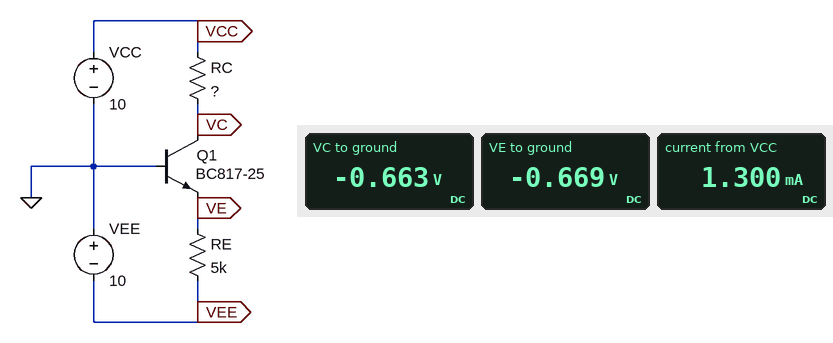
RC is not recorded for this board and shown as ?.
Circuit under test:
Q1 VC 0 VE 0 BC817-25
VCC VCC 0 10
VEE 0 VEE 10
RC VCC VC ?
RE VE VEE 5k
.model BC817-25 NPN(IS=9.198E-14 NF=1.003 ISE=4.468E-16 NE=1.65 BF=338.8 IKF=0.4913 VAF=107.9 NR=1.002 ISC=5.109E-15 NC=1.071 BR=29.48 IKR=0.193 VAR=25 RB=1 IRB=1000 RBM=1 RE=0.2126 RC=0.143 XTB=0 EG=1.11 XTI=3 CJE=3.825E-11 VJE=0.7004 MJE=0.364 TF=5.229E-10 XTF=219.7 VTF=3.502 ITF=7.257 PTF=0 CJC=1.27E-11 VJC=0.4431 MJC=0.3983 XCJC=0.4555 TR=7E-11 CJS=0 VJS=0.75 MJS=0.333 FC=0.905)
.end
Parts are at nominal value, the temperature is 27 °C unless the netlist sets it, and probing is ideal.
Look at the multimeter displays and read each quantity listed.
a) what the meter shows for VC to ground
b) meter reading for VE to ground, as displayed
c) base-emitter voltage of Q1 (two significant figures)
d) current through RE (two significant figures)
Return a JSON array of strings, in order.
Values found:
["-0.663 V", "-0.669 V", "670 mV", "1.9 mA"]
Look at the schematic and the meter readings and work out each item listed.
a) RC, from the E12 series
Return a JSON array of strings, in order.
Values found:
["8.2 kΩ"]
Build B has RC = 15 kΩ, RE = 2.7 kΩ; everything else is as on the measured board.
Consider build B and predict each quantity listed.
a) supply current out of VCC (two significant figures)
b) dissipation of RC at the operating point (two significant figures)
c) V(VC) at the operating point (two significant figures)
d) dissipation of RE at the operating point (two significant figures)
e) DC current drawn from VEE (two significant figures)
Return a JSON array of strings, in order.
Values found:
["710 µA", "7.6 mW", "-710 mV", "32 mW", "3.4 mA"]
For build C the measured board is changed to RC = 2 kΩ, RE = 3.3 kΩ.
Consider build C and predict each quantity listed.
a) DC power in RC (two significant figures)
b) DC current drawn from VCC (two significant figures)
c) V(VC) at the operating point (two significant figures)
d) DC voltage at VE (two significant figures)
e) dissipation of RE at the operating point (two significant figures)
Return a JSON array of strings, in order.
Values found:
["16 mW", "2.8 mA", "4.3 V", "-630 mV", "27 mW"]
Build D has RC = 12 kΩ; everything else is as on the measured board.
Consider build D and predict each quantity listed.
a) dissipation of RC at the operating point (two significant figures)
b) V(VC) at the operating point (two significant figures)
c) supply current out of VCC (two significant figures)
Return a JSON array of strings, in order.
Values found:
["9.5 mW", "-680 mV", "890 µA"]
